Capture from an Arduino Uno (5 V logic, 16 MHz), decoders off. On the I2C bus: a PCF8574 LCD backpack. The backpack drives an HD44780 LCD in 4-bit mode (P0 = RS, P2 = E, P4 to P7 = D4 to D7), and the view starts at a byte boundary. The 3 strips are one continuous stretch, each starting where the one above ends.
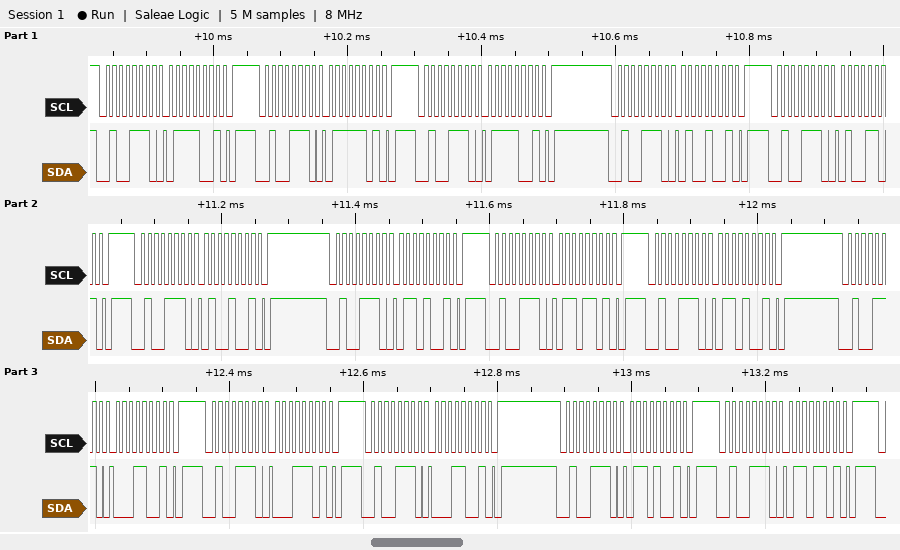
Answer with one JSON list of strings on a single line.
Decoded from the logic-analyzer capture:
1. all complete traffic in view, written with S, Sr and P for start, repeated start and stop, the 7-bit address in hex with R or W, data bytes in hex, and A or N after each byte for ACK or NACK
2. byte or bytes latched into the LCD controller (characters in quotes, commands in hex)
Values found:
["S 27W A 79 A P S 27W A 7D A P S 27W A 79 A P S 27W A 49 A P S 27W A 4D A P S 27W A 49 A P S 27W A 69 A P S 27W A 6D A P S 27W A 69 A P S 27W A 19 A P S 27W A 1D A P S 27W A 19 A P S 27W A 69 A P S 27W A 6D A P", "'t' 'a'"]
